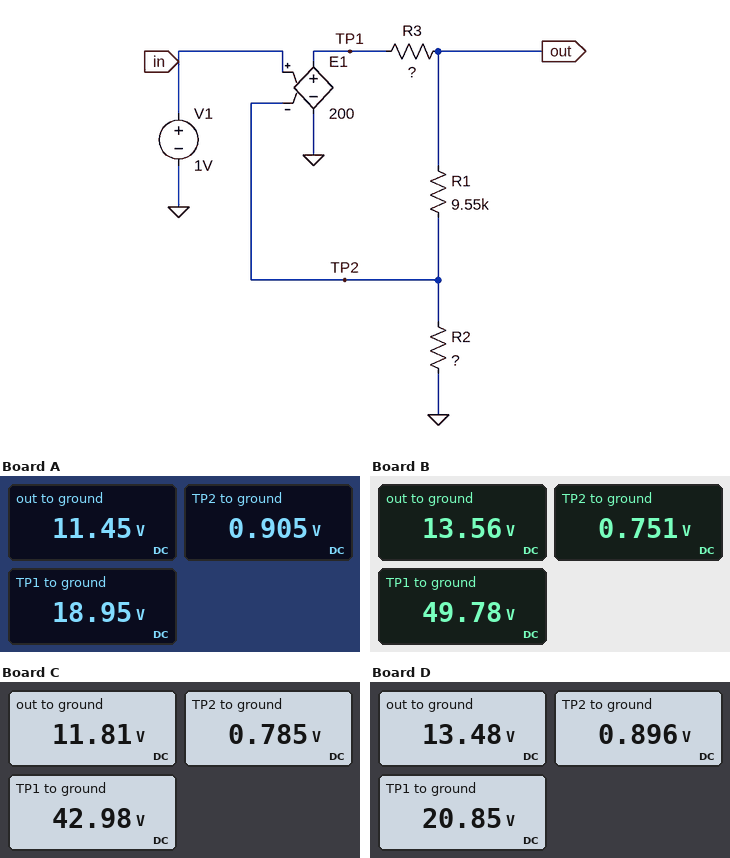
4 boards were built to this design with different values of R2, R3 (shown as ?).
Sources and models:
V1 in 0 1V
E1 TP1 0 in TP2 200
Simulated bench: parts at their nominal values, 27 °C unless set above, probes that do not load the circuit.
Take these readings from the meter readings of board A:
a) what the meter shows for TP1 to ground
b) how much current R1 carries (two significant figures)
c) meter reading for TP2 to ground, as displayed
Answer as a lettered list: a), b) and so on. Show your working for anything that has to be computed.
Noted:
a) 18.95 V
b) (11.45 V - 905 mV) / 9.55 kΩ = 1.1 mA
c) 0.905 V
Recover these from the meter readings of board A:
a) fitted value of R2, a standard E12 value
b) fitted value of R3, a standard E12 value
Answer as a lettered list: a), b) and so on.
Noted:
a) 820 Ω
b) 6.8 kΩ
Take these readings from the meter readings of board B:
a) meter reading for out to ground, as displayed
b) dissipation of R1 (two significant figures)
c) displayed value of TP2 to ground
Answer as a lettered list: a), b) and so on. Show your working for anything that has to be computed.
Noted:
a) 13.56 V
b) (13.56 V - 751 mV)^2 / 9.55 kΩ = 17 mW
c) 0.751 V
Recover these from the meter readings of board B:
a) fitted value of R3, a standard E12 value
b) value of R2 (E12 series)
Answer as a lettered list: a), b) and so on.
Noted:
a) 27 kΩ
b) 560 Ω
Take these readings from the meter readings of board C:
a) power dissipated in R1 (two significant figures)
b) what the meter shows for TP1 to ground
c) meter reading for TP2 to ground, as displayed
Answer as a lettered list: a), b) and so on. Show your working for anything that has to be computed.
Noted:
a) (11.81 V - 785 mV)^2 / 9.55 kΩ = 13 mW
b) 42.98 V
c) 0.785 V
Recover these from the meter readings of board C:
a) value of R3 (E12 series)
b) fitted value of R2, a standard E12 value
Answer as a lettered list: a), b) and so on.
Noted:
a) 27 kΩ
b) 680 Ω
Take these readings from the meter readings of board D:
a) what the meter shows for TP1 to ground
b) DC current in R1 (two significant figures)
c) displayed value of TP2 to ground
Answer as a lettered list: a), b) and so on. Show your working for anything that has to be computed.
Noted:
a) 20.85 V
b) (13.48 V - 896 mV) / 9.55 kΩ = 1.3 mA
c) 0.896 V
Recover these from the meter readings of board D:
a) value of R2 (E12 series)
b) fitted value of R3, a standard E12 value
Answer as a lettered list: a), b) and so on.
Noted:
a) 680 Ω
b) 5.6 kΩ
